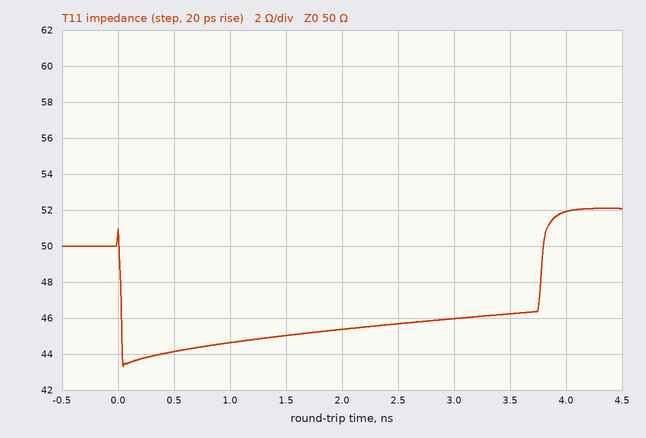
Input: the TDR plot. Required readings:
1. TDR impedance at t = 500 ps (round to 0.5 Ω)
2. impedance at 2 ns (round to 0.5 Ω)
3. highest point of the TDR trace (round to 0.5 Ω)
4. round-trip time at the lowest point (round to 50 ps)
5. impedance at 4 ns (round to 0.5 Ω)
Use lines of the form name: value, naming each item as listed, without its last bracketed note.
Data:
TDR impedance at t = 500 ps: 44.0 Ω
impedance at 2 ns: 45.5 Ω
highest point of the TDR trace: 52.0 Ω
round-trip time at the lowest point: 50 ps
impedance at 4 ns: 52.0 Ω
